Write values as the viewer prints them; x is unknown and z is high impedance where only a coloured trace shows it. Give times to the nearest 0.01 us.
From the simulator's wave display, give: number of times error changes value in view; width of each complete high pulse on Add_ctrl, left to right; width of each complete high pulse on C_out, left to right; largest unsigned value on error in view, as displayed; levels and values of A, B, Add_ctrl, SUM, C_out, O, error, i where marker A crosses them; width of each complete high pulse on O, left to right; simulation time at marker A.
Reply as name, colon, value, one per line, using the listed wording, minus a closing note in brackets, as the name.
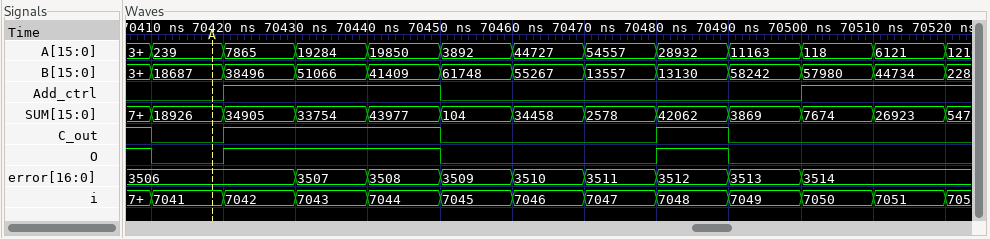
number of times error changes value in view: 8
width of each complete high pulse on Add_ctrl, left to right: 0.03 us
width of each complete high pulse on C_out, left to right: 0.03 us, 0.01 us
largest unsigned value on error in view, as displayed: 3514
levels and values of A, B, Add_ctrl, SUM, C_out, O, error, i where marker A crosses them: A=239, B=18687, Add_ctrl=0, SUM=18926, C_out=0, O=0, error=3506, i=7041
width of each complete high pulse on O, left to right: 0.03 us, 0.01 us
simulation time at marker A: 70.42 us
